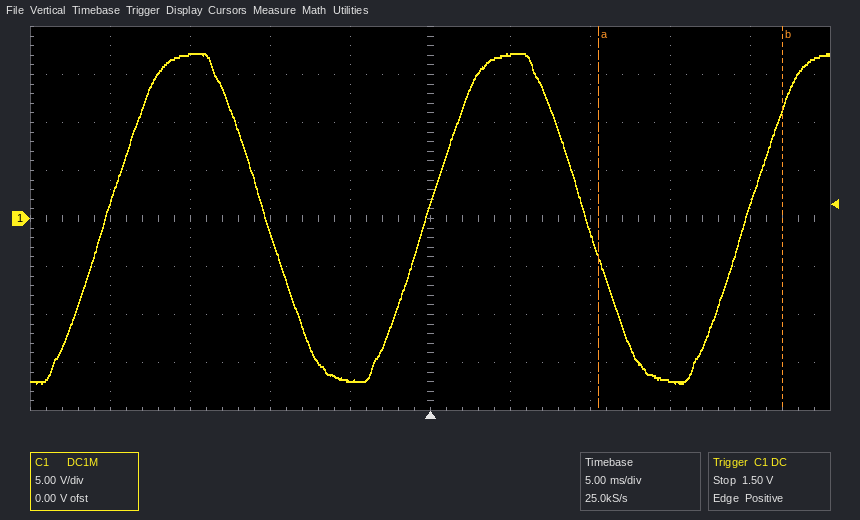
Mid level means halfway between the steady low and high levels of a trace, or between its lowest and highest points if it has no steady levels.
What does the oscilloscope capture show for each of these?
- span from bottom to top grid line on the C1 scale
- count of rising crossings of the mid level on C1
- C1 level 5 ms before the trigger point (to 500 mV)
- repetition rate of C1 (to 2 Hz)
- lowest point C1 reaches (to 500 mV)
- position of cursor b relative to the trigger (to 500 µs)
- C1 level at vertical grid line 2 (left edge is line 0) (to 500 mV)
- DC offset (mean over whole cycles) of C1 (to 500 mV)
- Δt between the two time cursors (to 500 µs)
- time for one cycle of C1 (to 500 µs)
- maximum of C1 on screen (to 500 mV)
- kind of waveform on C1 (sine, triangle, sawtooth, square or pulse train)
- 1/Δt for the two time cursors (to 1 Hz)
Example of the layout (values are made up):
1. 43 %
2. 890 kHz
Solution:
1. 40 V
2. 3
3. -17.0 V
4. 50 Hz
5. -17.0 V
6. +22.0 ms
7. 17.0 V
8. 0.0 V
9. 11.5 ms
10. 20.0 ms
11. 17.0 V
12. sine
13. 87 Hz
